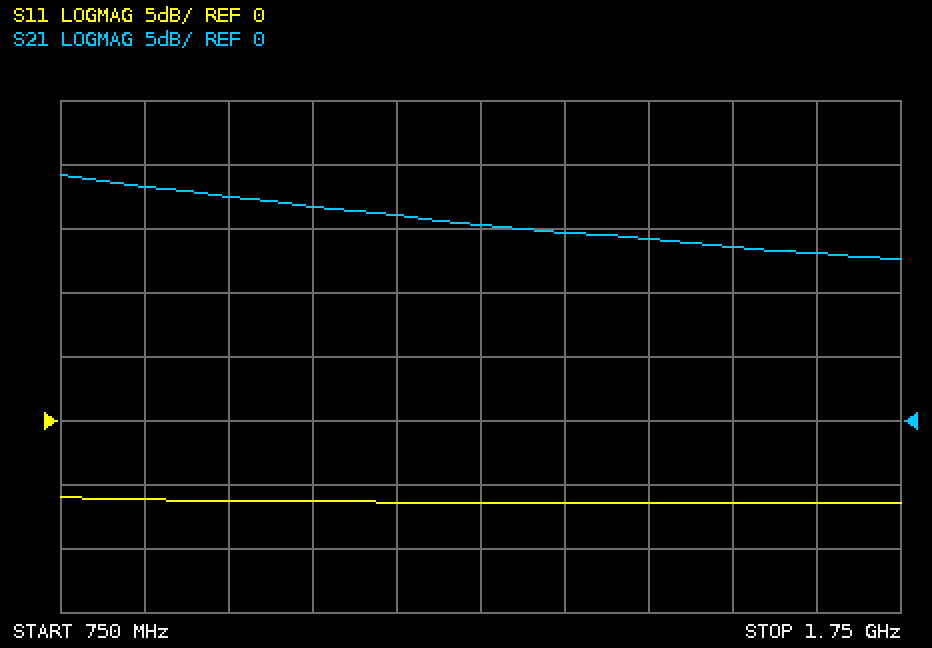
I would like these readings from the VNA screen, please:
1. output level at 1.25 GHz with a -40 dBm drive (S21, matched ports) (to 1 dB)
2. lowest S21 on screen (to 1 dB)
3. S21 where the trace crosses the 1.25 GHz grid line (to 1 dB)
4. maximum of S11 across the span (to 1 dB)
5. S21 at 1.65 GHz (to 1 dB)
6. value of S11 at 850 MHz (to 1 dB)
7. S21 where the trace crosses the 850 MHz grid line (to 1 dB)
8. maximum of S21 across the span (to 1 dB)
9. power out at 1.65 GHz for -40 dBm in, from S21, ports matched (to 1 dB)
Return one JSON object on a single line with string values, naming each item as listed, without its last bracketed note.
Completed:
{"output level at 1.25 GHz with a -40 dBm drive (S21, matched ports)": "-25 dBm", "lowest S21 on screen": "13 dB", "S21 where the trace crosses the 1.25 GHz grid line": "15 dB", "maximum of S11 across the span": "-6 dB", "S21 at 1.65 GHz": "13 dB", "value of S11 at 850 MHz": "-6 dB", "S21 where the trace crosses the 850 MHz grid line": "18 dB", "maximum of S21 across the span": "19 dB", "power out at 1.65 GHz for -40 dBm in, from S21, ports matched": "-27 dBm"}
